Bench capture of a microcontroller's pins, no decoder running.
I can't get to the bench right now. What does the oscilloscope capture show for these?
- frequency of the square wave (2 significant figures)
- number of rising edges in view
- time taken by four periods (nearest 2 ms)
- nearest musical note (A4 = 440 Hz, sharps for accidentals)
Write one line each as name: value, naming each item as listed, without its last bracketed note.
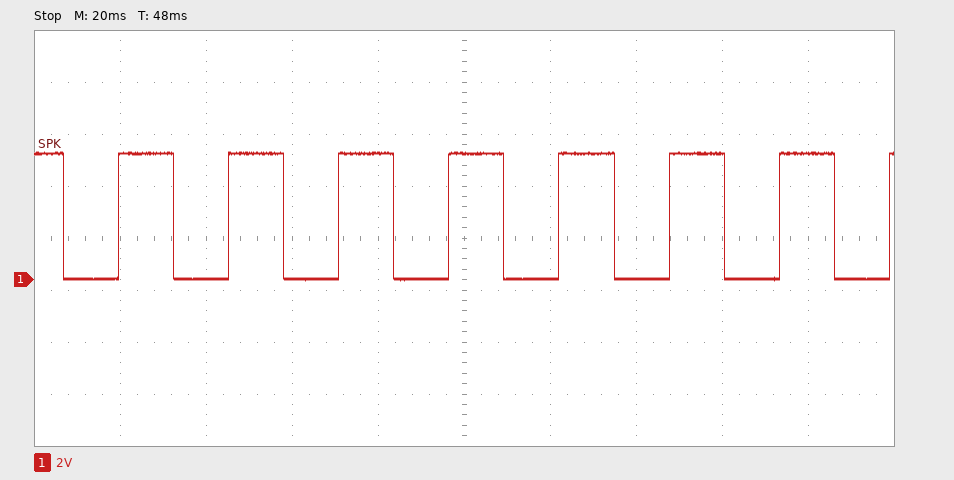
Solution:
frequency of the square wave: 39 Hz
number of rising edges in view: 8
time taken by four periods: 102 ms
nearest musical note: D#1
